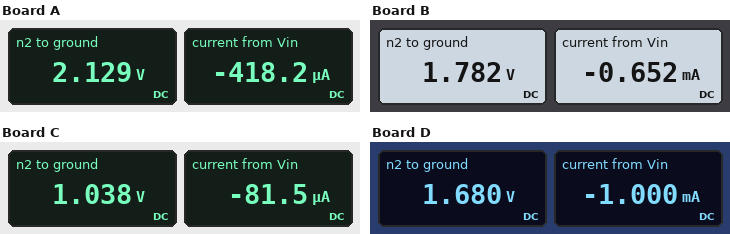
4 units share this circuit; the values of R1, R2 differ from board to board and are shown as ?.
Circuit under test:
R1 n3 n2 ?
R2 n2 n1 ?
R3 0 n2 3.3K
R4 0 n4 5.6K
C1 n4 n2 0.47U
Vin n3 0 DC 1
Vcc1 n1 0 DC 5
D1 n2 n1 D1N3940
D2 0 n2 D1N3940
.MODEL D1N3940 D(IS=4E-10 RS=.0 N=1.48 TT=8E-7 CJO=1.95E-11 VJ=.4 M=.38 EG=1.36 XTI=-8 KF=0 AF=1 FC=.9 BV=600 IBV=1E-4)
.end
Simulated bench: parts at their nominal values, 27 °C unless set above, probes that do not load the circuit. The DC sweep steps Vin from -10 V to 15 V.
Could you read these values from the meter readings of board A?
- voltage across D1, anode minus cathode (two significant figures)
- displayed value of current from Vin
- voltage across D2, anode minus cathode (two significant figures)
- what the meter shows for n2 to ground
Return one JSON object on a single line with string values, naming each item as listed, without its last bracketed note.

{"voltage across D1, anode minus cathode": "-2.9 V", "displayed value of current from Vin": "-418.2 µA", "voltage across D2, anode minus cathode": "-2.1 V", "what the meter shows for n2 to ground": "2.129 V"}
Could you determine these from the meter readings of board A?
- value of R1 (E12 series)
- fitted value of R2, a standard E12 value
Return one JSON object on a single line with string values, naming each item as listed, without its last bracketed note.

{"value of R1": "2.7 kΩ", "fitted value of R2, a standard E12 value": "2.7 kΩ"}
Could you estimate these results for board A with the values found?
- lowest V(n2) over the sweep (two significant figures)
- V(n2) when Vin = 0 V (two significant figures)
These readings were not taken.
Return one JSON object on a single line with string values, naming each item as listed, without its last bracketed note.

{"lowest V(n2) over the sweep": "-570 mV", "V(n2) when Vin = 0 V": "1.8 V"}
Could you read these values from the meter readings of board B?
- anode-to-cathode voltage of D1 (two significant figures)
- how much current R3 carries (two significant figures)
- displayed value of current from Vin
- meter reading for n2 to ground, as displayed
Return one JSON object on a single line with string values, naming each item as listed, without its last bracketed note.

{"anode-to-cathode voltage of D1": "-3.2 V", "how much current R3 carries": "540 µA", "displayed value of current from Vin": "-0.652 mA", "meter reading for n2 to ground, as displayed": "1.782 V"}
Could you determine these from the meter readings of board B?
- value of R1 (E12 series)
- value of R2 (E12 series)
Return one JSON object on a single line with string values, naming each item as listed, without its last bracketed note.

{"value of R1": "1.2 kΩ", "value of R2": "2.7 kΩ"}
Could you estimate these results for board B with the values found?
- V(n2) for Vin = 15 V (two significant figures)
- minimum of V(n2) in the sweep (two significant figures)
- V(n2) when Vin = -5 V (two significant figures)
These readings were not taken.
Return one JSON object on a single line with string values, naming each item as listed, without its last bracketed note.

{"V(n2) for Vin = 15 V": "5.6 V", "minimum of V(n2) in the sweep": "-630 mV", "V(n2) when Vin = -5 V": "-580 mV"}
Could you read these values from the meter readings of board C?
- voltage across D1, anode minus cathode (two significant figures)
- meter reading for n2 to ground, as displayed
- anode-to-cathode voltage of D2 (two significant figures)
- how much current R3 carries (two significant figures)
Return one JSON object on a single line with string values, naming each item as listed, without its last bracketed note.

{"voltage across D1, anode minus cathode": "-4.0 V", "meter reading for n2 to ground, as displayed": "1.038 V", "anode-to-cathode voltage of D2": "-1.0 V", "how much current R3 carries": "310 µA"}
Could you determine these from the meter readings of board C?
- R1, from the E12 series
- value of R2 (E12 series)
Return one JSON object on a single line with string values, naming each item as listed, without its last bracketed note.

{"R1, from the E12 series": "470 Ω", "value of R2": "10 kΩ"}
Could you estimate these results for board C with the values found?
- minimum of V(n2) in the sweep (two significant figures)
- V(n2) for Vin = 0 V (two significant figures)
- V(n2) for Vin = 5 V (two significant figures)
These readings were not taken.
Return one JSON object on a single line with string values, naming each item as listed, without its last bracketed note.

{"minimum of V(n2) in the sweep": "-680 mV", "V(n2) for Vin = 0 V": "200 mV", "V(n2) for Vin = 5 V": "4.4 V"}
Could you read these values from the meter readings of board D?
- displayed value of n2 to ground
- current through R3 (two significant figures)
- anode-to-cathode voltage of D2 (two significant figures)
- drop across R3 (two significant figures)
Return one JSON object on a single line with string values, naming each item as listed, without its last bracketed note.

{"displayed value of n2 to ground": "1.680 V", "current through R3": "510 µA", "anode-to-cathode voltage of D2": "-1.7 V", "drop across R3": "1.7 V"}
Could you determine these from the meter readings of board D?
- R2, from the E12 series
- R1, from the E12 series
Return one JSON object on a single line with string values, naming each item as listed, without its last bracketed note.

{"R2, from the E12 series": "2.2 kΩ", "R1, from the E12 series": "680 Ω"}
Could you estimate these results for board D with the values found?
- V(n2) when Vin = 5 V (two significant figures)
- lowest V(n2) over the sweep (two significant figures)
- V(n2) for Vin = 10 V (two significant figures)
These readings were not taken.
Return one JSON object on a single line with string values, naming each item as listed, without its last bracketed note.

{"V(n2) when Vin = 5 V": "4.3 V", "lowest V(n2) over the sweep": "-660 mV", "V(n2) for Vin = 10 V": "5.6 V"}
